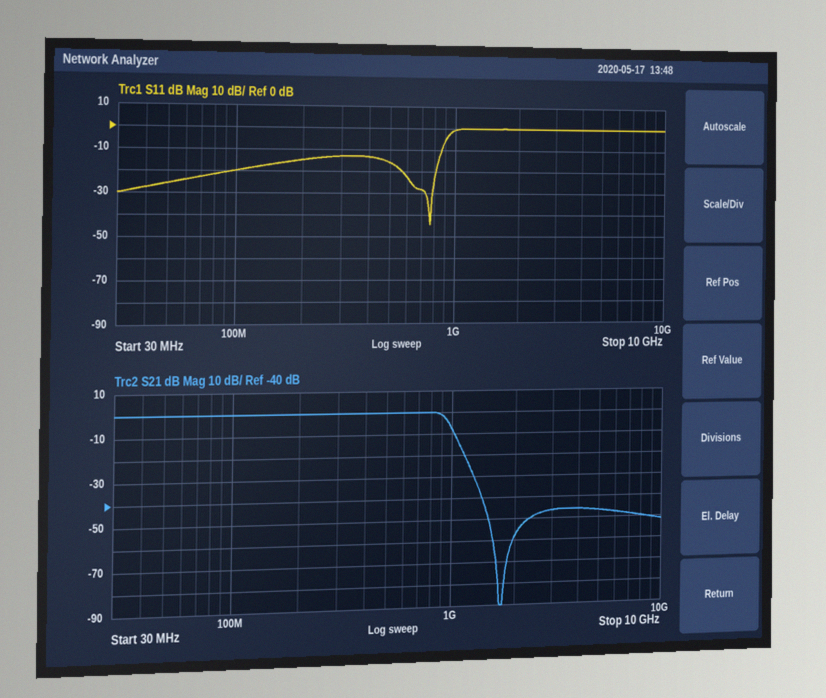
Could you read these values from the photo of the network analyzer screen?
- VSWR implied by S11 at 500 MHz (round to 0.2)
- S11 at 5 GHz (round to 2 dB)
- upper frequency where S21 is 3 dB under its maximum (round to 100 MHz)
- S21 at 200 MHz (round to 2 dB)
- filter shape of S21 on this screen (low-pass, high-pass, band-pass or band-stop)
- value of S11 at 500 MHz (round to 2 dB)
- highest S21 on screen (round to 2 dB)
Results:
1.4
0 dB
900 MHz
0 dB
low-pass
-16 dB
0 dB
